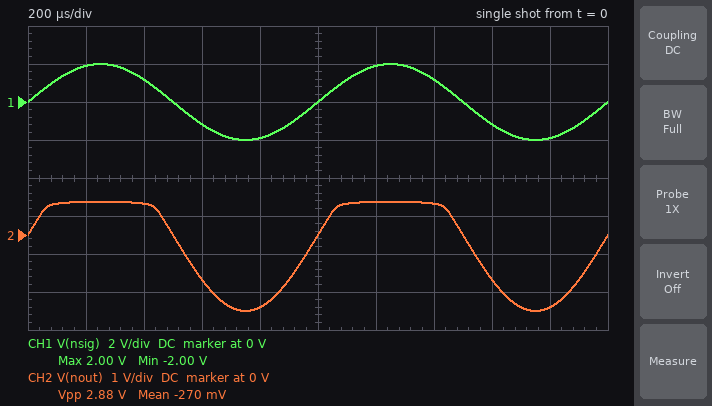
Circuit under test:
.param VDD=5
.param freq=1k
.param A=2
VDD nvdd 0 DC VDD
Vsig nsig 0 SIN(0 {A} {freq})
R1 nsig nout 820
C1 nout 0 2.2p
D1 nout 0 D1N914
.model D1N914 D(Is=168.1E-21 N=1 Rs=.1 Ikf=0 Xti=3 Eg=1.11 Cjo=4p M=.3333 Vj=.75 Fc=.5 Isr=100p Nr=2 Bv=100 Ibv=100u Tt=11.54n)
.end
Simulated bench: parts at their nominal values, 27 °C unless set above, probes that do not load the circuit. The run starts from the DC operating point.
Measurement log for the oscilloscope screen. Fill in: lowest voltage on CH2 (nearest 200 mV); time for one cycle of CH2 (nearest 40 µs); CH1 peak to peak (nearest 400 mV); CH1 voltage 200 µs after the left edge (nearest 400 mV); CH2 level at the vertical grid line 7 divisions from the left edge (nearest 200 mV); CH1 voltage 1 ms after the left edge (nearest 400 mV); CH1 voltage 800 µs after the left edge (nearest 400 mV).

-2.0 V
1.00 ms
4.0 V
2.0 V
800 mV
0 V
-2.0 V
